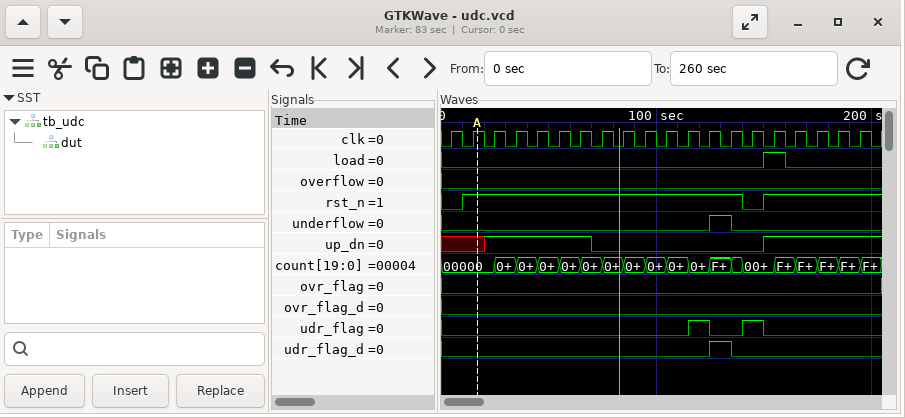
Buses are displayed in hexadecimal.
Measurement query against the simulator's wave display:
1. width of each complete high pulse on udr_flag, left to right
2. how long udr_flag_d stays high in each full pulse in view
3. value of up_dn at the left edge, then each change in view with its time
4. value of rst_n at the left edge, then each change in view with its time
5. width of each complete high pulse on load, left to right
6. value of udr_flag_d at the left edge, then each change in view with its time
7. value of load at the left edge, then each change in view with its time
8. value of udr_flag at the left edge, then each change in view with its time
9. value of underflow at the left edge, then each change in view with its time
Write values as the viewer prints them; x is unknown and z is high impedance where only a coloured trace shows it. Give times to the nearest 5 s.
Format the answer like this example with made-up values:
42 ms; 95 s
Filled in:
10 s, 10 s; 10 s; x, 1 at 20 s, 0 at 70 s, 1 at 150 s; 0, 1 at 10 s, 0 at 140 s, 1 at 150 s; 10 s; 0, 1 at 125 s, 0 at 135 s; 0, 1 at 150 s, 0 at 160 s; 0, 1 at 115 s, 0 at 125 s, 1 at 140 s, 0 at 150 s; 0, 1 at 125 s, 0 at 135 s
